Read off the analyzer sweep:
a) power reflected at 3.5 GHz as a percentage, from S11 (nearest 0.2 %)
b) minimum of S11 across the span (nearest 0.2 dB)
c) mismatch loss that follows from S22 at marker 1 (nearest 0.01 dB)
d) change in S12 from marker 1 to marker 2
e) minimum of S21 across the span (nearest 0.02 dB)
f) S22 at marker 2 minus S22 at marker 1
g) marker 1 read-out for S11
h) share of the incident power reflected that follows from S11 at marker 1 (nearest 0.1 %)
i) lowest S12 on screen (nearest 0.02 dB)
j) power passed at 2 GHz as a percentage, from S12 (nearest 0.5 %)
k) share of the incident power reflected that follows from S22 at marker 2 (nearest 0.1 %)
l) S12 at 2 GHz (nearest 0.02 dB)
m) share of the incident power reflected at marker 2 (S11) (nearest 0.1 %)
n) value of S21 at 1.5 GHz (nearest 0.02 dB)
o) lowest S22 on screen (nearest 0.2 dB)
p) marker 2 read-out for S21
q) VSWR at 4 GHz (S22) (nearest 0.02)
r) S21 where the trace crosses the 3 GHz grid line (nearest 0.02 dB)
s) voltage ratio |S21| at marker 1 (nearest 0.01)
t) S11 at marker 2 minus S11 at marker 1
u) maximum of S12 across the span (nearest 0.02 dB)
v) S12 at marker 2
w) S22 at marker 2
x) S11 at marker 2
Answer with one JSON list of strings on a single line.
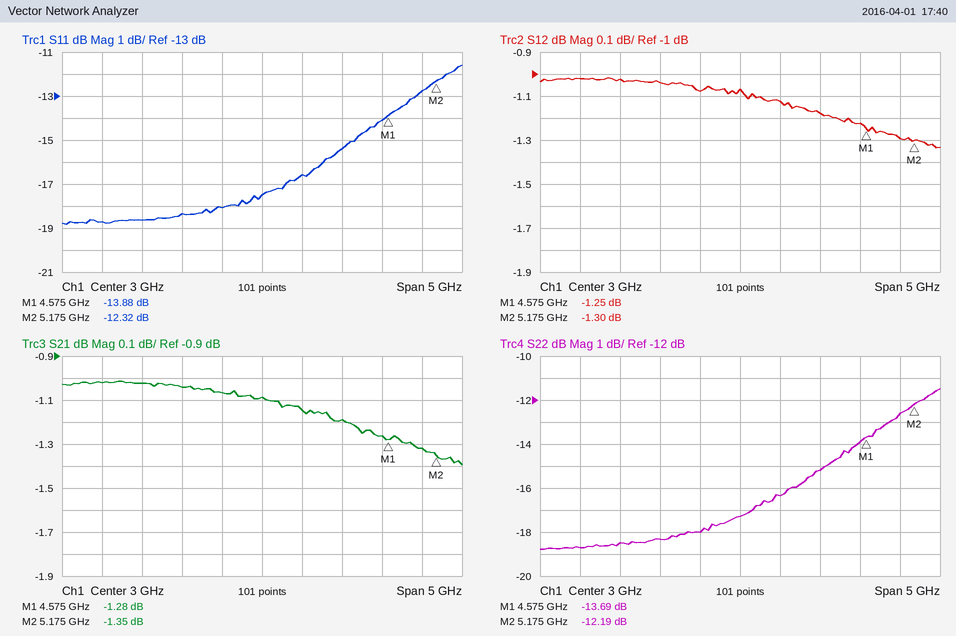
["2.2 %", "-18.8 dB", "0.19 dB", "-0.05 dB", "-1.40 dB", "1.50 dB", "-13.88 dB", "4.1 %", "-1.34 dB", "78.5 %", "6.0 %", "-1.04 dB", "5.9 %", "-1.02 dB", "-18.8 dB", "-1.35 dB", "1.42", "-1.08 dB", "0.86", "1.56 dB", "-1.02 dB", "-1.30 dB", "-12.19 dB", "-12.32 dB"]
